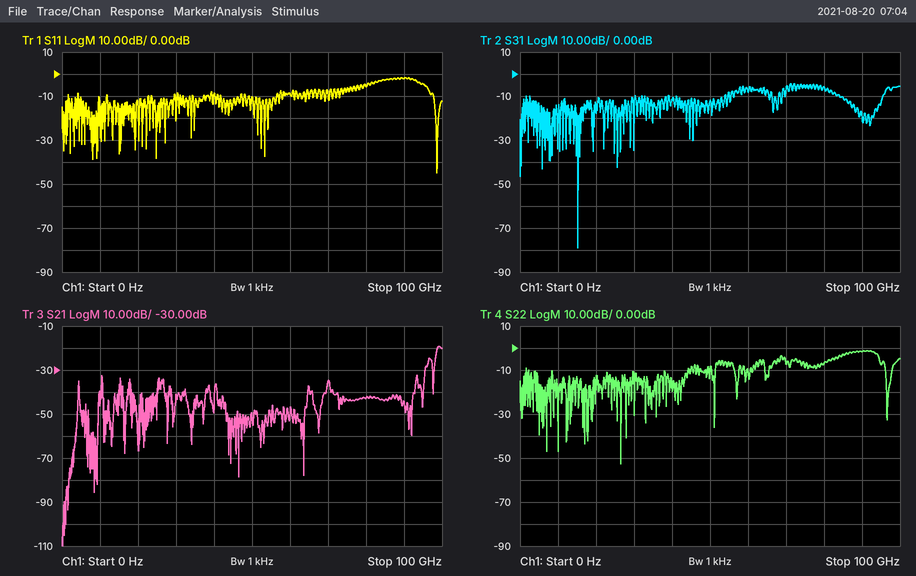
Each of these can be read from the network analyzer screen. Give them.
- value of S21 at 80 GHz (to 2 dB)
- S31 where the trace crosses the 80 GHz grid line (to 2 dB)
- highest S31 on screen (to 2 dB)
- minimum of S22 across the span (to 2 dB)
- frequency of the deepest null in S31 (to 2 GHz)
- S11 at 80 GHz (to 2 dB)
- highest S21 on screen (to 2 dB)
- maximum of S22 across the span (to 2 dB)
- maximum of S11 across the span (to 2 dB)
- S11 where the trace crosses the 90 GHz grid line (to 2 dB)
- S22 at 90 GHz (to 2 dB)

-42 dB
-6 dB
-4 dB
-52 dB
16 GHz
-6 dB
-20 dB
-2 dB
-2 dB
-2 dB
-2 dB
